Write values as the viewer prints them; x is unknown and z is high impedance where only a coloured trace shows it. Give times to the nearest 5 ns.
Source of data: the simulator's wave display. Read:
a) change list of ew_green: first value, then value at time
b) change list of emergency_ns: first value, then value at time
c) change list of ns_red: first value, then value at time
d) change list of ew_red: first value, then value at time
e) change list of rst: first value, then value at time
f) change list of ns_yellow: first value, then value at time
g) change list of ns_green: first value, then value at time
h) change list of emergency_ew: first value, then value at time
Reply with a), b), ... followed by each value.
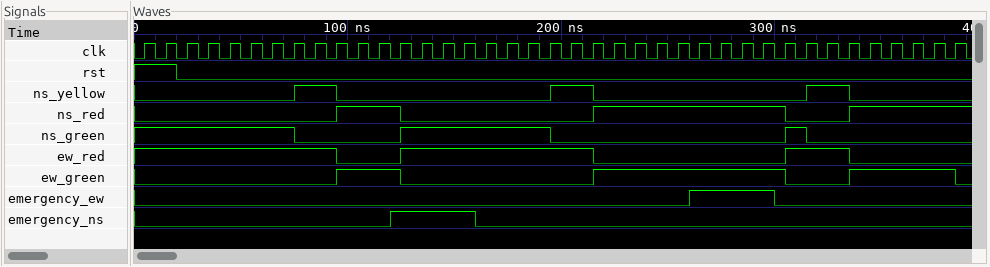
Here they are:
a) 0, 1 at 95 ns, 0 at 125 ns, 1 at 215 ns, 0 at 305 ns, 1 at 335 ns, 0 at 385 ns
b) 0, 1 at 120 ns, 0 at 160 ns
c) 0, 1 at 95 ns, 0 at 125 ns, 1 at 215 ns, 0 at 305 ns, 1 at 335 ns
d) 1, 0 at 95 ns, 1 at 125 ns, 0 at 215 ns, 1 at 305 ns, 0 at 335 ns
e) 1, 0 at 20 ns
f) 0, 1 at 75 ns, 0 at 95 ns, 1 at 195 ns, 0 at 215 ns, 1 at 315 ns, 0 at 335 ns
g) 1, 0 at 75 ns, 1 at 125 ns, 0 at 195 ns, 1 at 305 ns, 0 at 315 ns
h) 0, 1 at 260 ns, 0 at 300 ns
